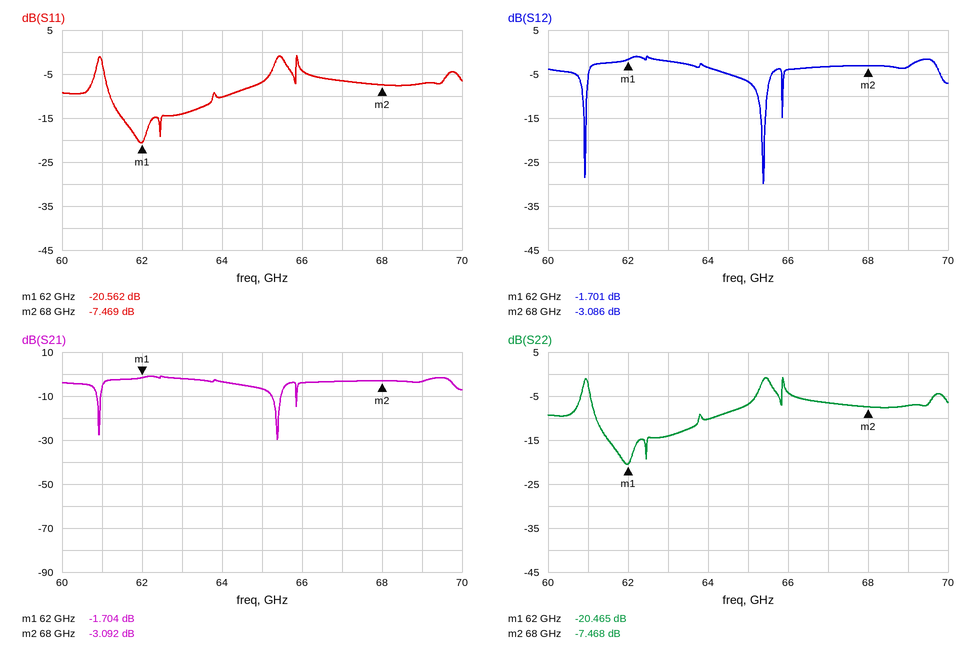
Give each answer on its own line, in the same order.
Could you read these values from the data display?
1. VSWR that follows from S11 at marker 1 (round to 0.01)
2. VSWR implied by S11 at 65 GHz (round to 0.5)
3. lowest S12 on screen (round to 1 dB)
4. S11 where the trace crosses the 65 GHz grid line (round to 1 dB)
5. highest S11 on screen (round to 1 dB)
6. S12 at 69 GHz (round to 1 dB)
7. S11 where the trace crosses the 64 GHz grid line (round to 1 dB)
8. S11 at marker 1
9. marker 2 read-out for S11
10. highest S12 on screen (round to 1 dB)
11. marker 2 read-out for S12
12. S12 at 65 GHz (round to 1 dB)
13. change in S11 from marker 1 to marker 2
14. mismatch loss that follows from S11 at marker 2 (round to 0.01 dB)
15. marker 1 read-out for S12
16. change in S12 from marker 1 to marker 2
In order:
1.21
2.5
-30 dB
-7 dB
-1 dB
-3 dB
-10 dB
-20.562 dB
-7.469 dB
-1 dB
-3.086 dB
-7 dB
13.093 dB
0.86 dB
-1.701 dB
-1.385 dB
